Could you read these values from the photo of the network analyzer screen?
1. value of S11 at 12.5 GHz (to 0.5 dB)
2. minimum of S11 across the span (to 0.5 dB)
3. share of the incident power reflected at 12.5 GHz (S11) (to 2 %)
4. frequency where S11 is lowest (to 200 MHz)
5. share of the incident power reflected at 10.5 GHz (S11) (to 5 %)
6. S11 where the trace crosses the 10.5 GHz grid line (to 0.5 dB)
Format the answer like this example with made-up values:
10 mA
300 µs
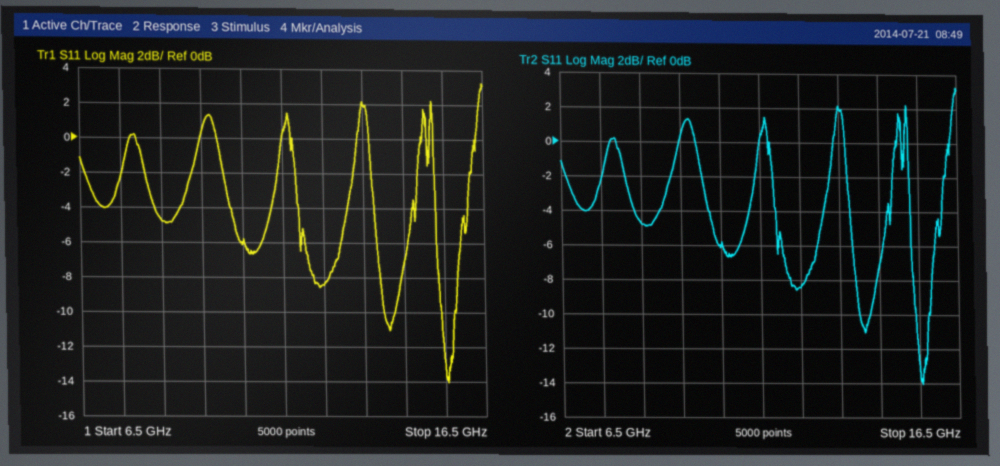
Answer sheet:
-8.5 dB
-14.0 dB
14 %
15.6 GHz
25 %
-6.0 dB
